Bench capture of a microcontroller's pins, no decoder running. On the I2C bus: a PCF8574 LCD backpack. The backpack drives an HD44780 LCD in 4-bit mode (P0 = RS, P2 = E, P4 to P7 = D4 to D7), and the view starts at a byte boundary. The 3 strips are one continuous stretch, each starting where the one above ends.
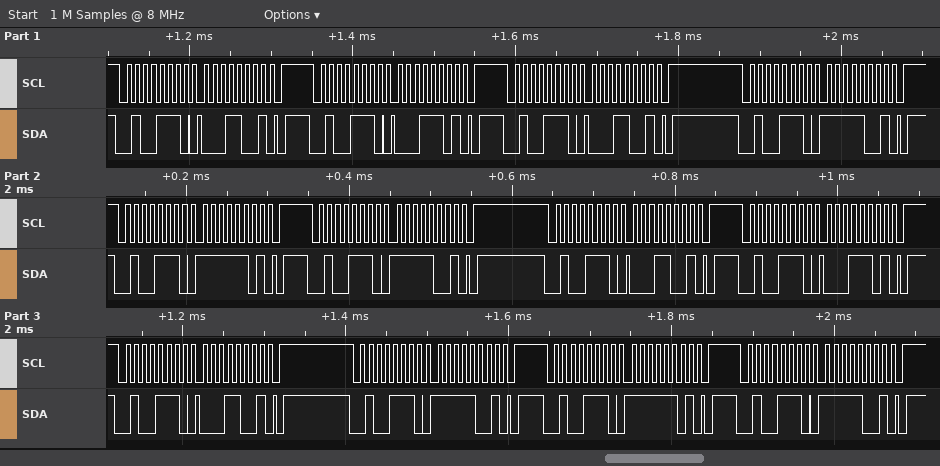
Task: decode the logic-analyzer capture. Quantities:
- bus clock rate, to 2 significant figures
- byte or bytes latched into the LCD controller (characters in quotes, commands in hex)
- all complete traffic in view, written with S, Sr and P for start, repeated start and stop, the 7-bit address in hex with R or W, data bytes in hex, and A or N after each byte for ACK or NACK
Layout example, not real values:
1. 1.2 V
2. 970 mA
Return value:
1. 100 kHz
2. data 0x1F data 0x1F
3. S 27W A 19 A P S 27W A 1D A P S 27W A 19 A P S 27W A F9 A P S 27W A FD A P S 27W A F9 A P S 27W A 19 A P S 27W A 1D A P S 27W A 19 A P S 27W A F9 A P S 27W A FD A P S 27W A F9 A P
